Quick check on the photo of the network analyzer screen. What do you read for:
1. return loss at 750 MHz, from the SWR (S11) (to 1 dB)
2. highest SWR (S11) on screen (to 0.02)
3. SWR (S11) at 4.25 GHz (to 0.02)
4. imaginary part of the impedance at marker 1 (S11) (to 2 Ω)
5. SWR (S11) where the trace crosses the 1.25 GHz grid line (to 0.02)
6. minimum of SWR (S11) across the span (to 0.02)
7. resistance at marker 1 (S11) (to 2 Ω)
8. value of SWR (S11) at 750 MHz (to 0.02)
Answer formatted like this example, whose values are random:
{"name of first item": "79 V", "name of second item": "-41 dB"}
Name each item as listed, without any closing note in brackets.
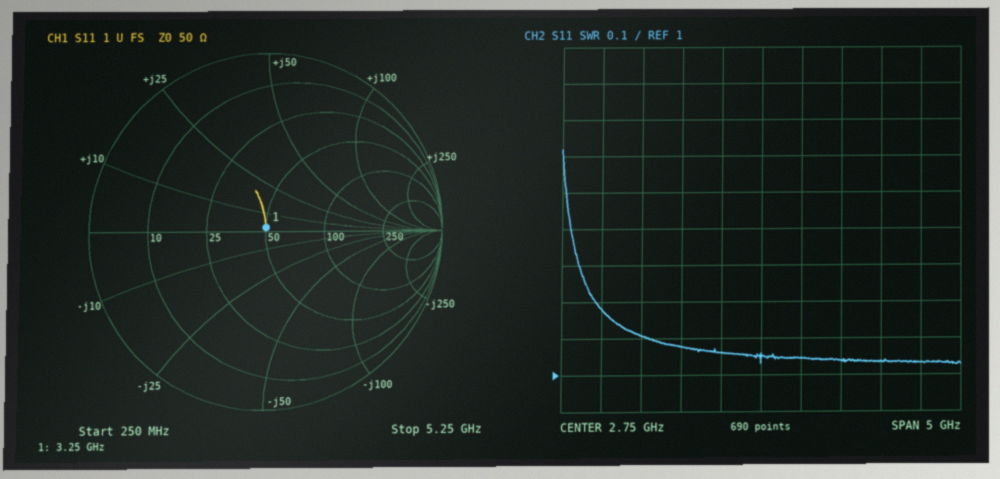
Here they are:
{"return loss at 750 MHz, from the SWR (S11)": "22 dB", "highest SWR (S11) on screen": "1.62", "SWR (S11) at 4.25 GHz": "1.04", "imaginary part of the impedance at marker 1 (S11)": "+2 Ω", "SWR (S11) where the trace crosses the 1.25 GHz grid line": "1.10", "minimum of SWR (S11) across the span": "1.02", "resistance at marker 1 (S11)": "50 Ω", "value of SWR (S11) at 750 MHz": "1.18"}
